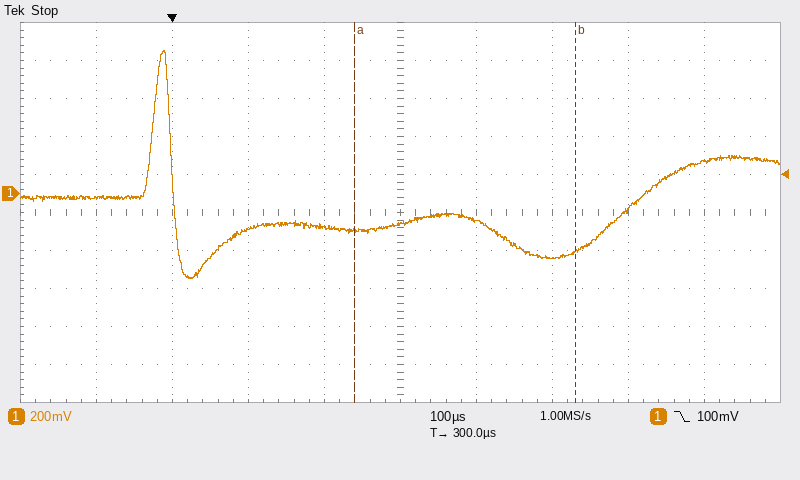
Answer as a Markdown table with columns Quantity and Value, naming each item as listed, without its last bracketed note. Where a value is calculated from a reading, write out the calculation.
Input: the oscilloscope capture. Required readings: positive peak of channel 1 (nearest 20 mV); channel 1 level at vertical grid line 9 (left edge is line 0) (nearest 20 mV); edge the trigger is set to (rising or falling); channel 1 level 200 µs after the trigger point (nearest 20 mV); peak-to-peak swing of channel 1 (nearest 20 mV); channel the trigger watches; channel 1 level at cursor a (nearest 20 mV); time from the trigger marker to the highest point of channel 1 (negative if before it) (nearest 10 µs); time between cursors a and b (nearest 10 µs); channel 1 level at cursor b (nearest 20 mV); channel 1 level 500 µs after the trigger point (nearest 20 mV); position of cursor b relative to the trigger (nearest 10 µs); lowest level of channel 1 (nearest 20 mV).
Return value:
| Quantity | Value |
|---|---|
| positive peak of channel 1 | 760 mV |
| channel 1 level at vertical grid line 9 (left edge is line 0) | 160 mV |
| edge the trigger is set to | falling |
| channel 1 level 200 µs after the trigger point | -180 mV |
| peak-to-peak swing of channel 1 | 760 mV − (-440 mV) = 1.20 V |
| channel the trigger watches | channel 1 |
| channel 1 level at cursor a | -200 mV |
| time from the trigger marker to the highest point of channel 1 (negative if before it) | -10 µs |
| time between cursors a and b | 290 µs |
| channel 1 level at cursor b | -300 mV |
| channel 1 level 500 µs after the trigger point | -340 mV |
| position of cursor b relative to the trigger | +530 µs |
| lowest level of channel 1 | -440 mV |
